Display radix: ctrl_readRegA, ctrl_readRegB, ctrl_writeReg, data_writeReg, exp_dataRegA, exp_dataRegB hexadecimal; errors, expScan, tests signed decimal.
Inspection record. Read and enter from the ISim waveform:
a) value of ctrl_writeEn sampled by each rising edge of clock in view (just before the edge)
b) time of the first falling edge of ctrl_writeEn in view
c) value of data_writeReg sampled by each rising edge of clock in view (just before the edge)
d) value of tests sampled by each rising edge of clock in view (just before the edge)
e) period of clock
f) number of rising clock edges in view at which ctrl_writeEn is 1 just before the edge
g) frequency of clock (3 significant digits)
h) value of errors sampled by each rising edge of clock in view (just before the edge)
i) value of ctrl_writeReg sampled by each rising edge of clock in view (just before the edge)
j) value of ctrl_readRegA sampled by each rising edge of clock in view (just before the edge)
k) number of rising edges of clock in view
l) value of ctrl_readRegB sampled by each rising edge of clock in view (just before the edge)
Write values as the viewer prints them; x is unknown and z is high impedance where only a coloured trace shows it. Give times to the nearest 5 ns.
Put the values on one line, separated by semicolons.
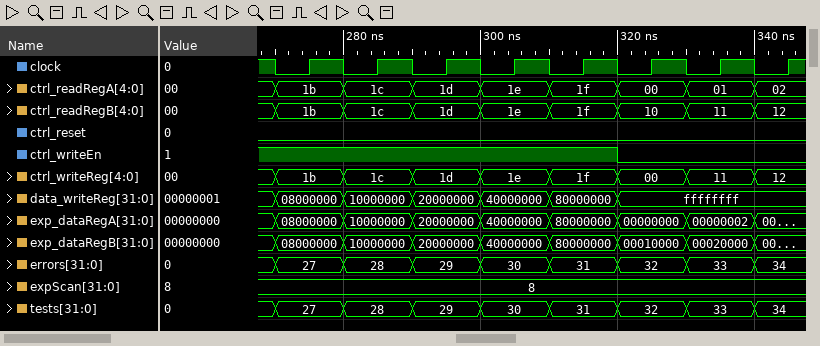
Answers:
1 1 1 1 1 0 0 0; 320 ns; 08000000, 10000000, 20000000, 40000000, 80000000, ffffffff, ffffffff, ffffffff; 27, 28, 29, 30, 31, 32, 33, 34; 10 ns; 5; 100 MHz; 27, 28, 29, 30, 31, 32, 33, 34; 1b, 1c, 1d, 1e, 1f, 00, 11, 12; 1b, 1c, 1d, 1e, 1f, 00, 01, 02; 8; 1b, 1c, 1d, 1e, 1f, 10, 11, 12
